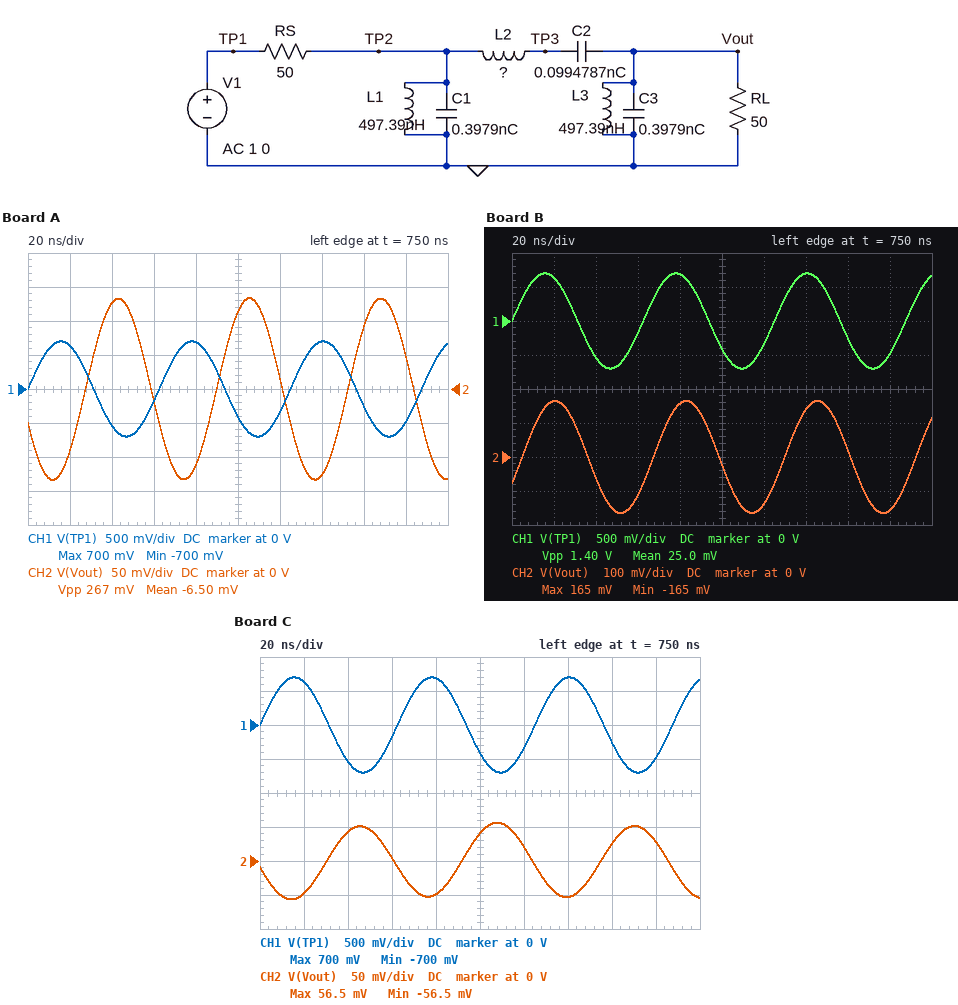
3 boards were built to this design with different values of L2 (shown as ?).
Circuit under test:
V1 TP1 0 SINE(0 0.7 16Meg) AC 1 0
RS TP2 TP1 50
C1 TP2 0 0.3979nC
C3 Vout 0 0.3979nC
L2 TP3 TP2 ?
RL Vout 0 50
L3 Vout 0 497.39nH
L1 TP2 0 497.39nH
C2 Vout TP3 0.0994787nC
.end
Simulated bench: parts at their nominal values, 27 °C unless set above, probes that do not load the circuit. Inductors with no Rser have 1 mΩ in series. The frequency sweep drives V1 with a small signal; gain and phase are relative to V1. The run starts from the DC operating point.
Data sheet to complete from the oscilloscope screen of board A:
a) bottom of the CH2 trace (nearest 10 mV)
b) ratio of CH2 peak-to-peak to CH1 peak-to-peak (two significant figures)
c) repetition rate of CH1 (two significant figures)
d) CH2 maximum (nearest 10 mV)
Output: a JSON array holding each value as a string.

["-130 mV", "0.19", "16 MHz", "130 mV"]
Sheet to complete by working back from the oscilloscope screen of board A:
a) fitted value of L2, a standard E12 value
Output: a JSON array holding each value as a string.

["2.7 µH"]
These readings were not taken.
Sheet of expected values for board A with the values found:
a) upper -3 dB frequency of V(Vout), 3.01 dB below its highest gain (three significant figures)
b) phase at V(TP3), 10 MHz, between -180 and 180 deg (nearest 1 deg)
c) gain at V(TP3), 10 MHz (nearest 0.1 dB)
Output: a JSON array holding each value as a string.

["13.8 MHz", "-78 deg", "3.3 dB"]
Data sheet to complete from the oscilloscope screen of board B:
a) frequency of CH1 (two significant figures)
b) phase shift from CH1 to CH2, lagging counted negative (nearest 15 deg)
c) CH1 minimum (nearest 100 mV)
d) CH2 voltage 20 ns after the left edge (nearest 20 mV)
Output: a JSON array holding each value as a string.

["16 MHz", "-30 deg", "-700 mV", "160 mV"]
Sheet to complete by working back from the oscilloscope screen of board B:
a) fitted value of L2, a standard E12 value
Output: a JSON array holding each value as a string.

["560 nH"]
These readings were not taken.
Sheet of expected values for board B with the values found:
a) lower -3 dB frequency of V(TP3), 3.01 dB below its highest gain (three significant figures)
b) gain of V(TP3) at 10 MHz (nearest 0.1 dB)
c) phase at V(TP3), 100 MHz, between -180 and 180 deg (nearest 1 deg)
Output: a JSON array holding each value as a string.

["24.6 MHz", "0.9 dB", "96 deg"]
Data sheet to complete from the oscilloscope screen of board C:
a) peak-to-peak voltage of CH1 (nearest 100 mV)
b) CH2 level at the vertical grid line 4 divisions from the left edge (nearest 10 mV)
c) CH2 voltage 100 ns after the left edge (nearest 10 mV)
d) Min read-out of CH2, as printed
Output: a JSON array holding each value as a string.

["1.4 V", "-50 mV", "40 mV", "-56.5 mV"]
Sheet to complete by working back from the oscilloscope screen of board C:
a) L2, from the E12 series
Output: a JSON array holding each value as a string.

["4.7 µH"]
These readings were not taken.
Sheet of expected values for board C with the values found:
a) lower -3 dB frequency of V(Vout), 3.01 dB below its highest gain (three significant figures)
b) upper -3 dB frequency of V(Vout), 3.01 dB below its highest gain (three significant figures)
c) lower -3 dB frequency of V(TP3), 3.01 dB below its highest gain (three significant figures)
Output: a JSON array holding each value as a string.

["6.30 MHz", "7.16 MHz", "6.22 MHz"]
